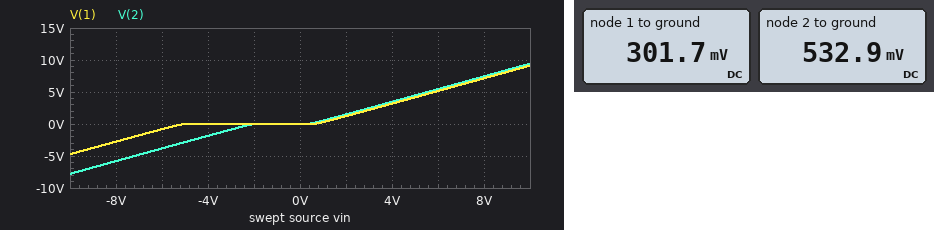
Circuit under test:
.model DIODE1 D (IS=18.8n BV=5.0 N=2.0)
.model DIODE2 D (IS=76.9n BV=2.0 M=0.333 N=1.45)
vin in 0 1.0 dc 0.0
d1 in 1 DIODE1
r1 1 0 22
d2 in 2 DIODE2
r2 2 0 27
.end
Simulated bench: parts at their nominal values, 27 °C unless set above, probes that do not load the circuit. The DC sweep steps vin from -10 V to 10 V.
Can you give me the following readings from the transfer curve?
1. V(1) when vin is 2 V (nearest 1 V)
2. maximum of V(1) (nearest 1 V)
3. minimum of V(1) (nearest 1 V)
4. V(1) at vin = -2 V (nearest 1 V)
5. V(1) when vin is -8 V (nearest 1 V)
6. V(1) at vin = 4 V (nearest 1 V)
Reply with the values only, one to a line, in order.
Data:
1 V
9 V
-5 V
0 V
-3 V
3 V
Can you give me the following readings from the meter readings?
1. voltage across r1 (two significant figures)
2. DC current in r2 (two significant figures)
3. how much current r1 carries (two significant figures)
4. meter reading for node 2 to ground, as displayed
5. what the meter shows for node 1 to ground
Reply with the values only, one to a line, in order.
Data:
300 mV
20 mA
14 mA
532.9 mV
301.7 mV
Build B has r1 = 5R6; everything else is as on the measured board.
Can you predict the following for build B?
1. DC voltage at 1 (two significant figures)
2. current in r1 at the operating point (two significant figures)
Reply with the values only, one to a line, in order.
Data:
240 mV
43 mA
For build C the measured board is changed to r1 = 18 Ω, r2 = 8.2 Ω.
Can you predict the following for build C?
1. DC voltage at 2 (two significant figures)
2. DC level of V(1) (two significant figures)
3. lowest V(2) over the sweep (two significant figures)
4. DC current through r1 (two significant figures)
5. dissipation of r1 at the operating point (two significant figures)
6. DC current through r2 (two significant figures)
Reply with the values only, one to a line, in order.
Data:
490 mV
290 mV
-7.7 V
16 mA
4.8 mW
60 mA
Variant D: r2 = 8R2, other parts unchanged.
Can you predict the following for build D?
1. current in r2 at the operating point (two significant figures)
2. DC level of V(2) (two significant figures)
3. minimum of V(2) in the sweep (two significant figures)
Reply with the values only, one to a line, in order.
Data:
60 mA
490 mV
-7.7 V
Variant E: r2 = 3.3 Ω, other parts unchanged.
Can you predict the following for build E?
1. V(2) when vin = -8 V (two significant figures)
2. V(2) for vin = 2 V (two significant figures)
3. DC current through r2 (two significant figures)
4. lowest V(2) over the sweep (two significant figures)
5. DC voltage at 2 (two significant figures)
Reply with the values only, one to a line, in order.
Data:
-5.7 V
1.4 V
140 mA
-7.7 V
460 mV
